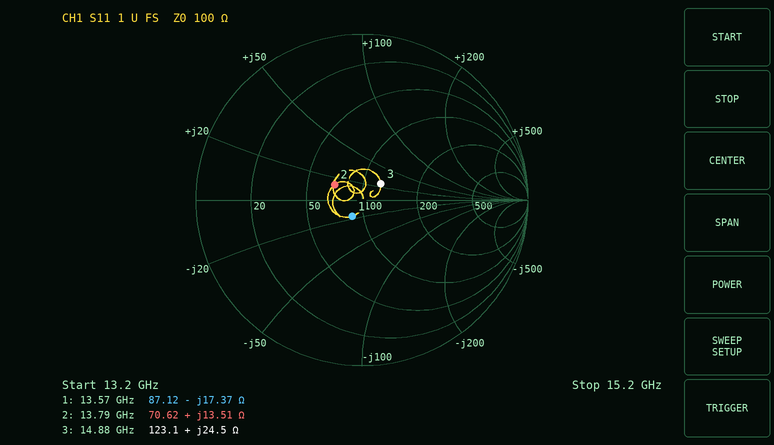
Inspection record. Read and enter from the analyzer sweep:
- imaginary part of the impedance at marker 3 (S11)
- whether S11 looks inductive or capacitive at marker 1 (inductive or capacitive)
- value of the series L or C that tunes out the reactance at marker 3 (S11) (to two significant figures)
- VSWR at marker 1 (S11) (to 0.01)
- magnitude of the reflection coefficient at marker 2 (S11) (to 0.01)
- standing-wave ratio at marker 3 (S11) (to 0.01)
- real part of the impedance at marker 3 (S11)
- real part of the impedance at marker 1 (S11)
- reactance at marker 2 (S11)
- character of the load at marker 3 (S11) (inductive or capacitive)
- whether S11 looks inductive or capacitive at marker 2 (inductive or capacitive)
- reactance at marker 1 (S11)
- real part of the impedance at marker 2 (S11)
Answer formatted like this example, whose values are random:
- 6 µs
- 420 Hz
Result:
- +24.5 Ω
- capacitive
- 440 fF
- 1.26
- 0.19
- 1.35
- 123.1 Ω
- 87.12 Ω
- +13.51 Ω
- inductive
- inductive
- -17.37 Ω
- 70.62 Ω
